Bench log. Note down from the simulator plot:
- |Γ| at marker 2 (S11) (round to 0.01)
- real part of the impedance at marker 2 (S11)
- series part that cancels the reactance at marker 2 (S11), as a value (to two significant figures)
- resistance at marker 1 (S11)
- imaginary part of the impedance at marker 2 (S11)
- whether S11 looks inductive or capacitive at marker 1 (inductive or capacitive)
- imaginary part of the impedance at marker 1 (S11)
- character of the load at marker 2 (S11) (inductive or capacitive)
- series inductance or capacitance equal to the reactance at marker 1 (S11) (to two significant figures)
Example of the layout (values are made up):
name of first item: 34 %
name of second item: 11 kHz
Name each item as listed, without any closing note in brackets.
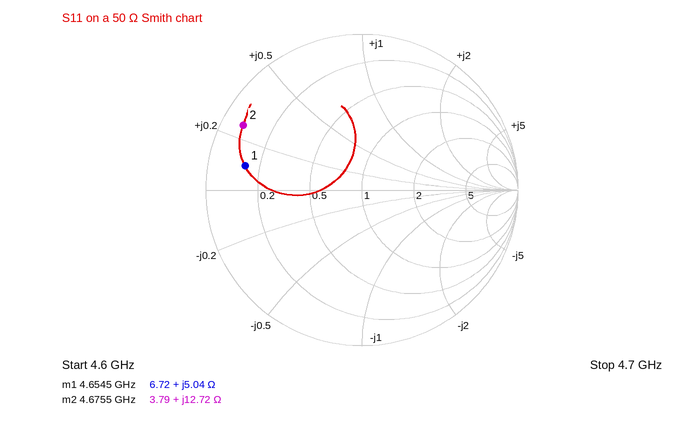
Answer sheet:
|Γ| at marker 2 (S11): 0.87
real part of the impedance at marker 2: 3.79 Ω
series part that cancels the reactance at marker 2 (S11), as a value: 2.7 pF
resistance at marker 1: 6.72 Ω
imaginary part of the impedance at marker 2: +12.72 Ω
whether S11 looks inductive or capacitive at marker 1: inductive
imaginary part of the impedance at marker 1: +5.04 Ω
character of the load at marker 2 (S11): inductive
series inductance or capacitance equal to the reactance at marker 1 (S11): 170 pH
